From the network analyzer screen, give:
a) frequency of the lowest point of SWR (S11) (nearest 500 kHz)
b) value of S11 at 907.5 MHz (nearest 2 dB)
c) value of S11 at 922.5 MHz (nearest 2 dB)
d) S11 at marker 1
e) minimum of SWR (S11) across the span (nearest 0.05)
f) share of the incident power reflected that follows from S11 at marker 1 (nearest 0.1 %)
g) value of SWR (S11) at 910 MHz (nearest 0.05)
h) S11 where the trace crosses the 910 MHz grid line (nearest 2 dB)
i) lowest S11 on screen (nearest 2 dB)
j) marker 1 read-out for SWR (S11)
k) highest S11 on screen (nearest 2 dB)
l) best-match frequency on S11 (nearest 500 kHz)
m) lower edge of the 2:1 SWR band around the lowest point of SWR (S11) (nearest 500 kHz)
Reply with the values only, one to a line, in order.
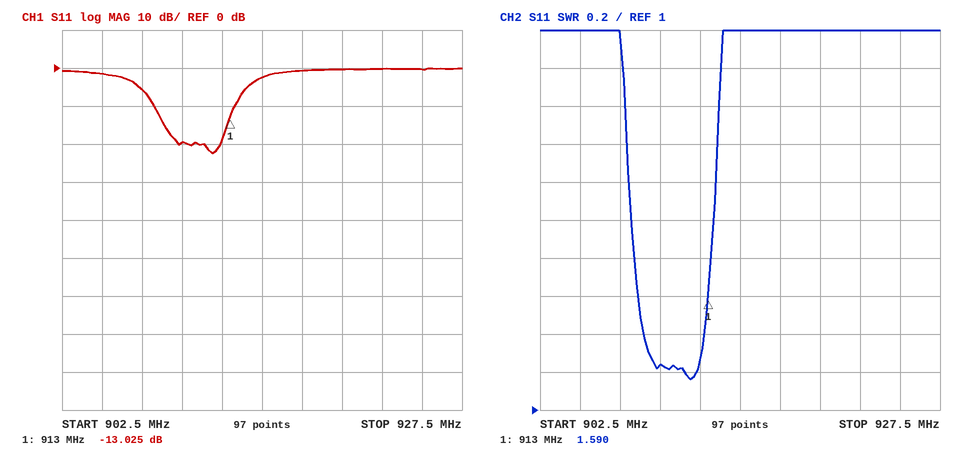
912.0 MHz
-6 dB
0 dB
-13.025 dB
1.15
5.0 %
1.25
-20 dB
-22 dB
1.590
0 dB
912.0 MHz
908.0 MHz
